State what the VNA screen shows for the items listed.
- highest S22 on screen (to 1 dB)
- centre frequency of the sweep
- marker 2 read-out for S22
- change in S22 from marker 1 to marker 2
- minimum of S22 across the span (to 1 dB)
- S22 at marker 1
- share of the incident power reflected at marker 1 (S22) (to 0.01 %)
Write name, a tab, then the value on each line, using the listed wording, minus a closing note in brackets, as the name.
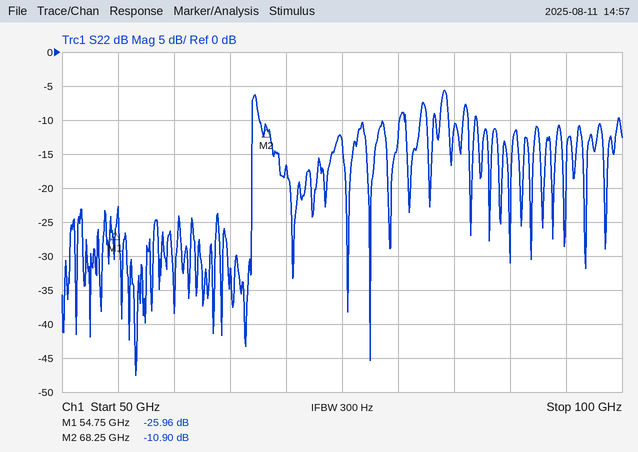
highest S22 on screen	-6 dB
centre frequency of the sweep	75 GHz
marker 2 read-out for S22	-10.90 dB
change in S22 from marker 1 to marker 2	15.06 dB
minimum of S22 across the span	-48 dB
S22 at marker 1	-25.96 dB
share of the incident power reflected at marker 1 (S22)	0.25 %
